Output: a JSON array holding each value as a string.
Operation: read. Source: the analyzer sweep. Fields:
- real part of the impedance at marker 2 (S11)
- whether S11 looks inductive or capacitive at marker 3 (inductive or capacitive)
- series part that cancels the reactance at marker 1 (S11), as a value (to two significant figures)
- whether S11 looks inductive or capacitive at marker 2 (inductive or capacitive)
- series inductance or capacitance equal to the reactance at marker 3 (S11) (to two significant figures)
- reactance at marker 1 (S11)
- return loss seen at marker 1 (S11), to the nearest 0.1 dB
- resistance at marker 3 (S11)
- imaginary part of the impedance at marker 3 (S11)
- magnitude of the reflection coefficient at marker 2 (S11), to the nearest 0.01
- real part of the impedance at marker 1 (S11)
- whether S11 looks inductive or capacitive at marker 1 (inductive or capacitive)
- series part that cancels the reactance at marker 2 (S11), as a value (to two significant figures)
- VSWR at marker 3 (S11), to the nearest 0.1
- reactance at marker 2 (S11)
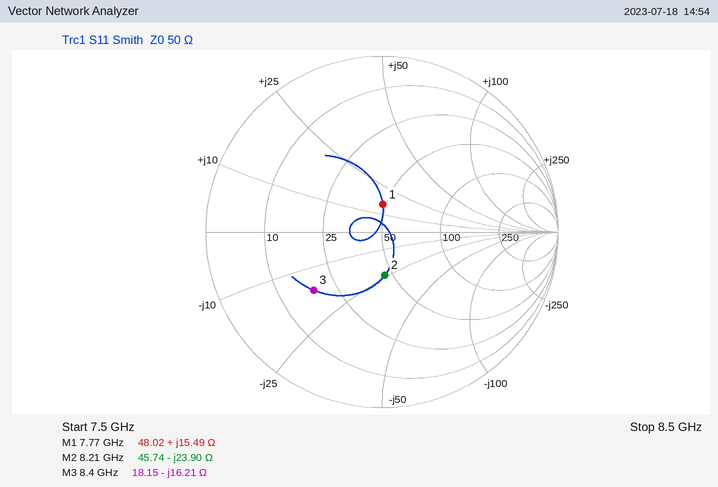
["45.74 Ω", "capacitive", "1.3 pF", "capacitive", "1.2 pF", "+15.49 Ω", "16.1 dB", "18.15 Ω", "-16.21 Ω", "0.25", "48.02 Ω", "inductive", "460 pH", "3.1", "-23.90 Ω"]
